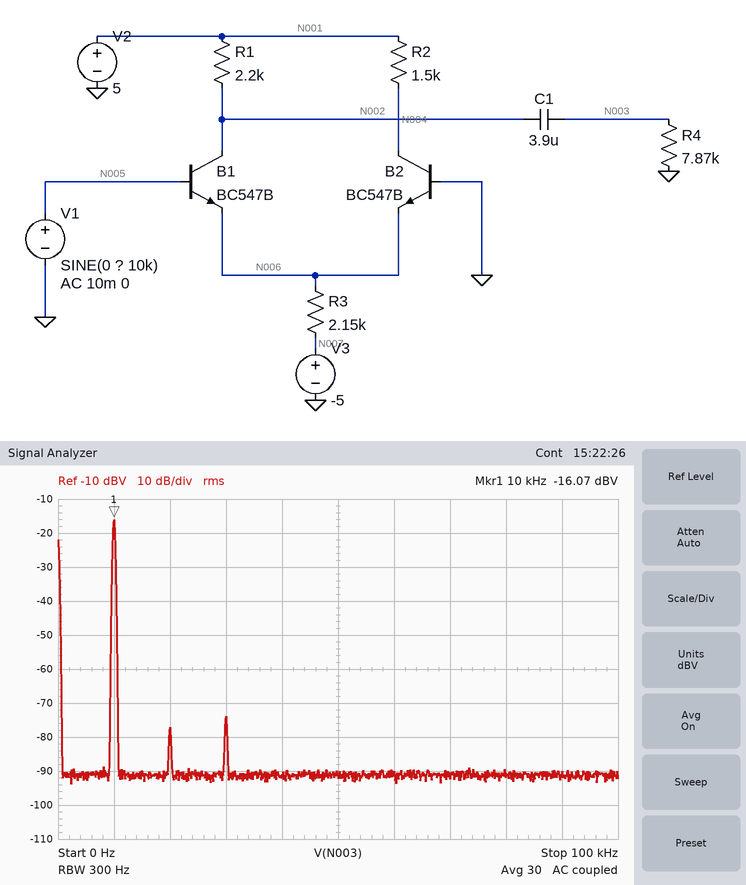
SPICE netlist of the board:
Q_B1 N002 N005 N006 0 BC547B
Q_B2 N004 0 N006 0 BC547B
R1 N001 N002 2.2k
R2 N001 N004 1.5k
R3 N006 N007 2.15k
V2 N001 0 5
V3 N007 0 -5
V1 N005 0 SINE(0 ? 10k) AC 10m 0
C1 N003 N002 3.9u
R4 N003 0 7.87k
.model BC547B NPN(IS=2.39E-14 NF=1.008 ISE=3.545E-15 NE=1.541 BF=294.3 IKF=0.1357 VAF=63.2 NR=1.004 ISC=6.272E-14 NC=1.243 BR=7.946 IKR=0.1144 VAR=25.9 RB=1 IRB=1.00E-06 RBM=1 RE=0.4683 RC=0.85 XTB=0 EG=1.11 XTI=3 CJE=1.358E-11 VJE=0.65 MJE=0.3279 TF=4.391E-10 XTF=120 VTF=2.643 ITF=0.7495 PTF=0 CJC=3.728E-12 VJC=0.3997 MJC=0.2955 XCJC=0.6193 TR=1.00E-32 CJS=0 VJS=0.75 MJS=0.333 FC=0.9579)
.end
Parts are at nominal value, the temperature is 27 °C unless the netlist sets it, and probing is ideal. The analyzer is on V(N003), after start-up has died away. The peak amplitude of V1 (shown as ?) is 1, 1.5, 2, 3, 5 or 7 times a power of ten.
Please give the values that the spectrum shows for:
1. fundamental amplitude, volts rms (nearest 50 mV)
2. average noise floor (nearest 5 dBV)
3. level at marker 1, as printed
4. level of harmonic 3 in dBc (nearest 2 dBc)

150 mV
-90 dBV
-16.07 dBV
-58 dBc
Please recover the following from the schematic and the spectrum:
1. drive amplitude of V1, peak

7 mV
